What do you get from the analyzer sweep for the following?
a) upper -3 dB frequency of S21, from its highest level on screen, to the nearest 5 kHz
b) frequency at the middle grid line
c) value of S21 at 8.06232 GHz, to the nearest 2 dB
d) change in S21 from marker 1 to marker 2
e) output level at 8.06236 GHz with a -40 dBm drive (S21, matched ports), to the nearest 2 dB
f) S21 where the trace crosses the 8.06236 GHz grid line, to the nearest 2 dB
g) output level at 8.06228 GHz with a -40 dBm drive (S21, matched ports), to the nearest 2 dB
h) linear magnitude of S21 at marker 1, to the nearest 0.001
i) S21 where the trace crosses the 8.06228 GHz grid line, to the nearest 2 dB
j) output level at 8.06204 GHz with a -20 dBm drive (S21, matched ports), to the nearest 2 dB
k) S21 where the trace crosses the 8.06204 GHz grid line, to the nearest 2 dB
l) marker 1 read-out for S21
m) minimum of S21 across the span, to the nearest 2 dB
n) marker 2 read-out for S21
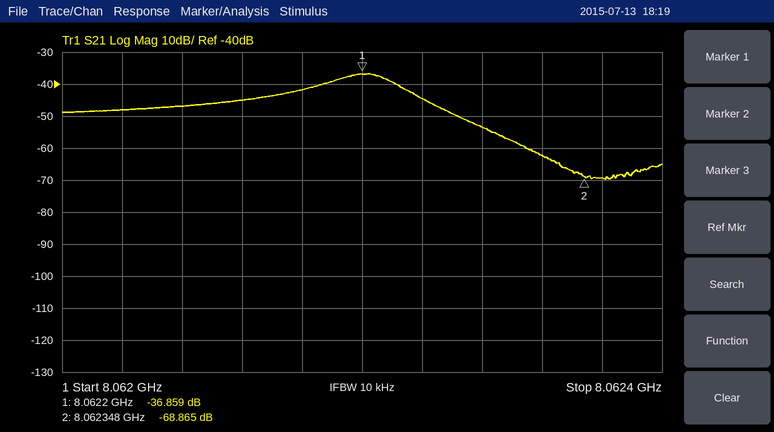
8.062220 GHz
8.0622 GHz
-62 dB
-32.006 dB
-110 dBm
-70 dB
-94 dBm
0.014
-54 dB
-68 dBm
-48 dB
-36.859 dB
-70 dB
-68.865 dB
